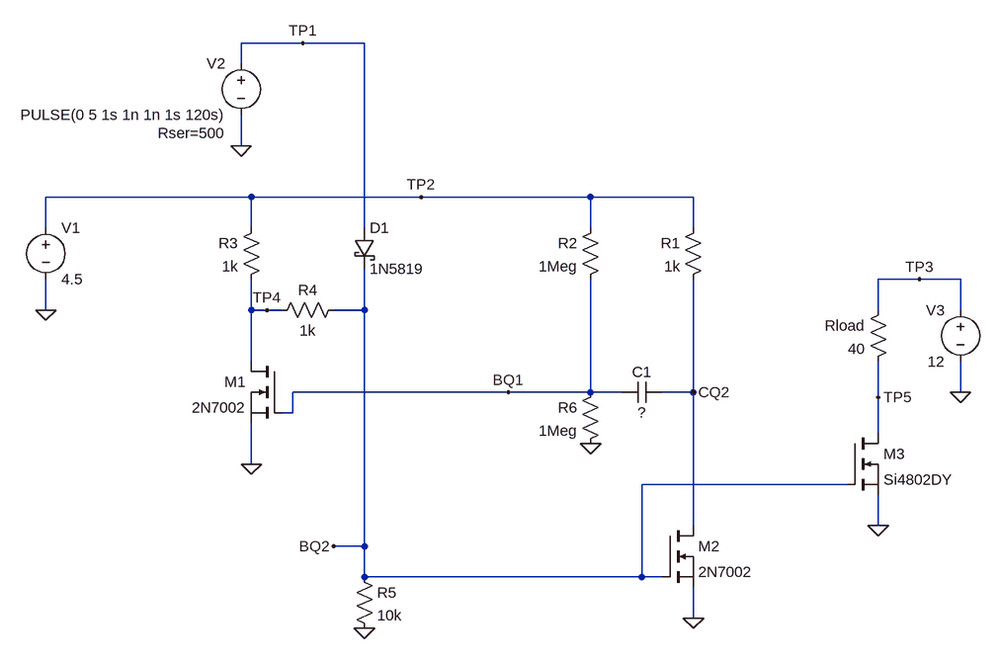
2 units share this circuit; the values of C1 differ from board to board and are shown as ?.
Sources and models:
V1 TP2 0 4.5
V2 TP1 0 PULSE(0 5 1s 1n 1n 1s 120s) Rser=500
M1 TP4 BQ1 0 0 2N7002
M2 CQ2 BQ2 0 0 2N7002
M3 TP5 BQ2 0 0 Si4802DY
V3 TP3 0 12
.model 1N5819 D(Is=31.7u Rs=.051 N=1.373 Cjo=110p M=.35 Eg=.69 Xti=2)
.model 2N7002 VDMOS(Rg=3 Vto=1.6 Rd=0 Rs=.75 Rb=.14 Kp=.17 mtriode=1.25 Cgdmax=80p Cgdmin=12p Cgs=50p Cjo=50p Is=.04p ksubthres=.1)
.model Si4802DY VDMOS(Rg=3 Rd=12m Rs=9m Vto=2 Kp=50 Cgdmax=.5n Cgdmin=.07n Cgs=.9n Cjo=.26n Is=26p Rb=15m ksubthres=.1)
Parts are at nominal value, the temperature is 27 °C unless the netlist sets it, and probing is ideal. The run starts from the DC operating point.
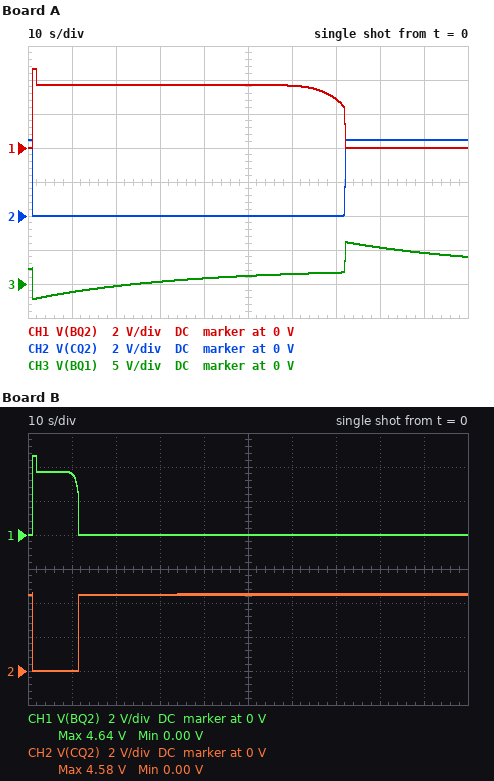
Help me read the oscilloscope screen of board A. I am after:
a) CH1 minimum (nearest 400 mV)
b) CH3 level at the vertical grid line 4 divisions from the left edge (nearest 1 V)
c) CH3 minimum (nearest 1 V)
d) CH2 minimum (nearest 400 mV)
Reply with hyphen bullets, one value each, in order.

- 0 V
- 1 V
- -2 V
- 0 V
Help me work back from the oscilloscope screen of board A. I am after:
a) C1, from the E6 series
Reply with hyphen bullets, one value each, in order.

- 68 µF
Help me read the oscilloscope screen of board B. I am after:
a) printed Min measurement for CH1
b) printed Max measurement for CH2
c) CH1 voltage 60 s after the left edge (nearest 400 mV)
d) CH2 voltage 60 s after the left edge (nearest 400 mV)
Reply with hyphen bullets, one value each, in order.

- 0.00 V
- 4.58 V
- 0 V
- 4.4 V
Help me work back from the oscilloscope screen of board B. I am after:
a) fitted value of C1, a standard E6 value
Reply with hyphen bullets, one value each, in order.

- 10 µF
